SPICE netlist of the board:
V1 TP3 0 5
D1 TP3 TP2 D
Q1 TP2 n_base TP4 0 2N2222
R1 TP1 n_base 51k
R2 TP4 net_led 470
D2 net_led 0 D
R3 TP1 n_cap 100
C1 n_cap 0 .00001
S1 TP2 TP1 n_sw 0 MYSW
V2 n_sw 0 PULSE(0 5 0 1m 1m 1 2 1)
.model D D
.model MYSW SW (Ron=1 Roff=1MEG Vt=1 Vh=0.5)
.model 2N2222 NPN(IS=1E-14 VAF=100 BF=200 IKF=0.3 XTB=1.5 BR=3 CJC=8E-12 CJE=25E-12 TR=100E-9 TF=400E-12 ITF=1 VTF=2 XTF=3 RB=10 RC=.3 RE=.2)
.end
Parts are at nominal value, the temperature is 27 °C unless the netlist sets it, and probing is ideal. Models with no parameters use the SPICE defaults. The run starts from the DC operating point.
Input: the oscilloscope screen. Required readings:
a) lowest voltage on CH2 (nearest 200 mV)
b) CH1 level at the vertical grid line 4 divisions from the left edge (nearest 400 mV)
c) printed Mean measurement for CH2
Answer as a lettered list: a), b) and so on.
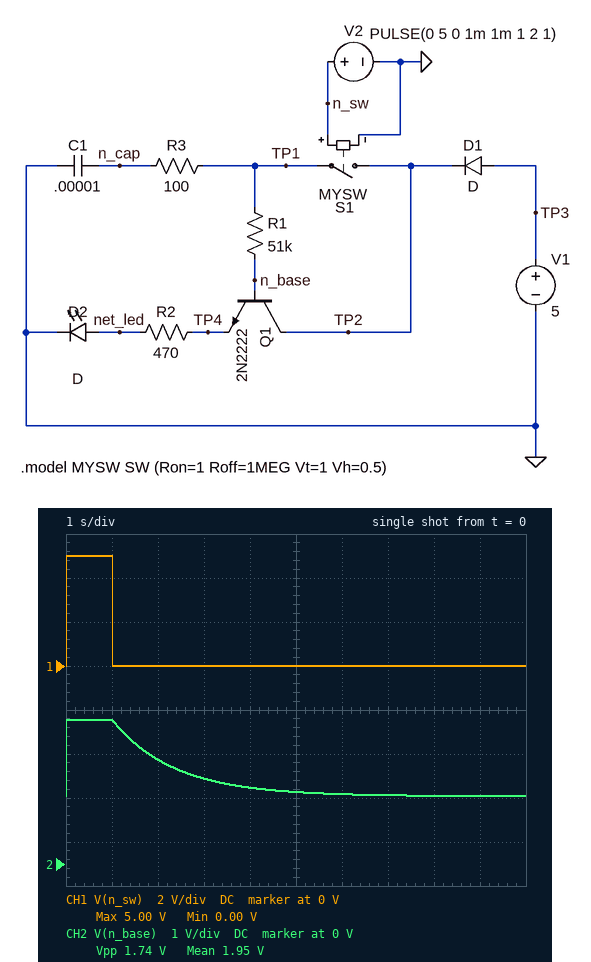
a) 1.6 V
b) 0 V
c) 1.95 V
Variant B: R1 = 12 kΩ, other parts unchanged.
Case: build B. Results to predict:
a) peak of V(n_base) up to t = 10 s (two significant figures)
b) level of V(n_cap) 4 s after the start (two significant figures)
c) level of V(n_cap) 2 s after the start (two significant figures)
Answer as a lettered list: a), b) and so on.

a) 4.0 V
b) 1.7 V
c) 2.6 V
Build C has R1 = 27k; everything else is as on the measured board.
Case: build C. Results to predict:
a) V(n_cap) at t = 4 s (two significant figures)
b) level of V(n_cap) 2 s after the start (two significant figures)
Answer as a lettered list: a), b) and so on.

a) 1.8 V
b) 2.7 V
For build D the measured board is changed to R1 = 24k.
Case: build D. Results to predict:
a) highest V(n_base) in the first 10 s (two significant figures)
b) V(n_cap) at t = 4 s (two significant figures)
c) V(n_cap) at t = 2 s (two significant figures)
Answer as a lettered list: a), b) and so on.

a) 3.7 V
b) 1.8 V
c) 2.7 V
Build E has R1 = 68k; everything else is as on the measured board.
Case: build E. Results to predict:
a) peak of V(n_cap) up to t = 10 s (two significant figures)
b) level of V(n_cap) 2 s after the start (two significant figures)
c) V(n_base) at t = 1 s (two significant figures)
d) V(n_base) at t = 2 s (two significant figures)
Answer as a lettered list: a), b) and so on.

a) 4.3 V
b) 3.0 V
c) 3.1 V
d) 2.3 V
